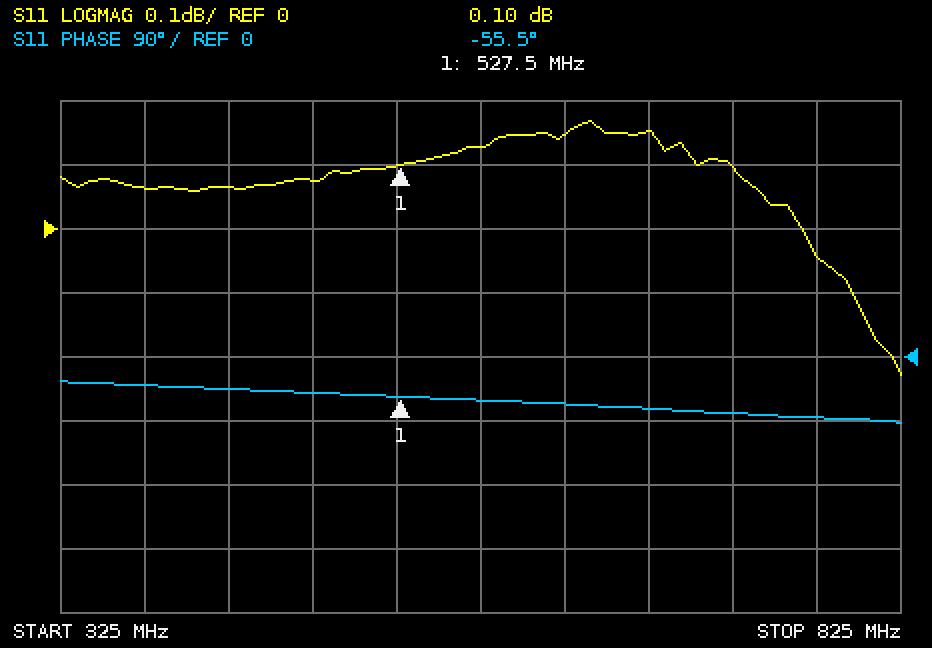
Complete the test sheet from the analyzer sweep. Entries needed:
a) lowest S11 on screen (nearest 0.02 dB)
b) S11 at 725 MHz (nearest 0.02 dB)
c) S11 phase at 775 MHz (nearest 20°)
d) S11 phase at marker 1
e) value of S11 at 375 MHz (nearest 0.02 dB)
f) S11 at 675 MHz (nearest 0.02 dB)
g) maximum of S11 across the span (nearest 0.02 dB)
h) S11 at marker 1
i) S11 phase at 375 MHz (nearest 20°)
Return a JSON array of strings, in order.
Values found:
["-0.22 dB", "0.10 dB", "-80°", "-55.5°", "0.06 dB", "0.16 dB", "0.16 dB", "0.10 dB", "-40°"]
